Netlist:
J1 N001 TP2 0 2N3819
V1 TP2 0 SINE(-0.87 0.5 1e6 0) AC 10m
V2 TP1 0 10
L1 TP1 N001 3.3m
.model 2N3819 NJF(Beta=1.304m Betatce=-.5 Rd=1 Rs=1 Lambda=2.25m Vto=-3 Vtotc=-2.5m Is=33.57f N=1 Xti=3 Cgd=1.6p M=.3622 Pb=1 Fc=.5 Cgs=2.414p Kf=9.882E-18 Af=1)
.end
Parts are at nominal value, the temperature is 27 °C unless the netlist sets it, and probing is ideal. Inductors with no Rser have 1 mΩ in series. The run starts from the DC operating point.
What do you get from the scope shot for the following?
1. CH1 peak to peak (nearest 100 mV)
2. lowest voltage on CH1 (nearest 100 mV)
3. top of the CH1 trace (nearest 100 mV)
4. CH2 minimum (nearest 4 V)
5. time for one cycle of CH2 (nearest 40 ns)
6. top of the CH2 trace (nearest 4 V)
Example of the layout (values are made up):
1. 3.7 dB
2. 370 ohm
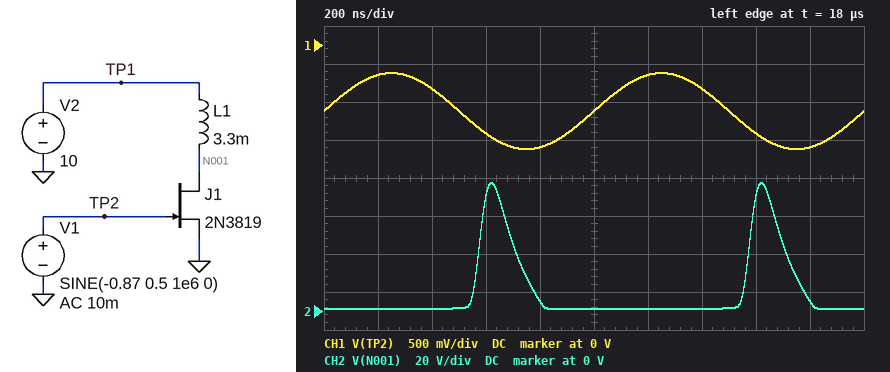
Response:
1. 1.0 V
2. -1.4 V
3. -400 mV
4. 0 V
5. 1.00 µs
6. 68 V
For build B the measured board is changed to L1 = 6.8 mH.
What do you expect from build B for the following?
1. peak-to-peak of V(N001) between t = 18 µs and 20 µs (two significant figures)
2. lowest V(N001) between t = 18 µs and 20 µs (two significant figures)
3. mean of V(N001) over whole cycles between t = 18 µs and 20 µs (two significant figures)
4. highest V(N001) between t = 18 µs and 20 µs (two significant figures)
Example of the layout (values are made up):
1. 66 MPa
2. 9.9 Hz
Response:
1. 70 V
2. 690 mV
3. 10 V
4. 71 V
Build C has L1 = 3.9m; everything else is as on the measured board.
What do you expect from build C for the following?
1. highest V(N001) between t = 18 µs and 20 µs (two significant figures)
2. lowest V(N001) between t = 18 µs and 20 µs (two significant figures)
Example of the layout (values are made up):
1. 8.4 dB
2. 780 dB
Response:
1. 69 V
2. 760 mV
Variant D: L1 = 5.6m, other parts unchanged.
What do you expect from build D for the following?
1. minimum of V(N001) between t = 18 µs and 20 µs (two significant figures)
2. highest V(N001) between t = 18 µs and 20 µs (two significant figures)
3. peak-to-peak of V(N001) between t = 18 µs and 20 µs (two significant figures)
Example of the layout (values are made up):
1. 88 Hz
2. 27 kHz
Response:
1. 700 mV
2. 71 V
3. 70 V
